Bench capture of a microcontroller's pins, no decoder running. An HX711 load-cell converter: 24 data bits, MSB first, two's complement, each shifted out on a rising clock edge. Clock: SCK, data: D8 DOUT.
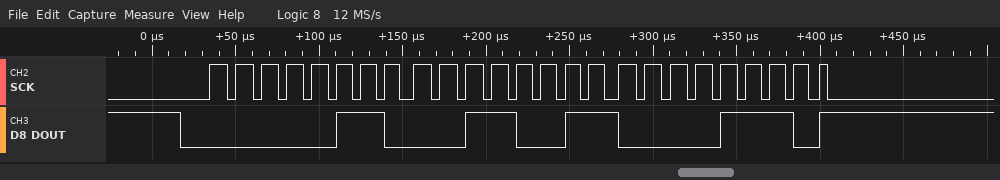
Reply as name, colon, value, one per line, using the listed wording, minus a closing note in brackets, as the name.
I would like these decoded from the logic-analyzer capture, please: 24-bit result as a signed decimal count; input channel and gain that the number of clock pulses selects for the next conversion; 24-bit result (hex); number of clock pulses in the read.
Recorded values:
24-bit result as a signed decimal count: 406286
input channel and gain that the number of clock pulses selects for the next conversion: channel A, gain 128
24-bit result: 0x06330E
number of clock pulses in the read: 25
